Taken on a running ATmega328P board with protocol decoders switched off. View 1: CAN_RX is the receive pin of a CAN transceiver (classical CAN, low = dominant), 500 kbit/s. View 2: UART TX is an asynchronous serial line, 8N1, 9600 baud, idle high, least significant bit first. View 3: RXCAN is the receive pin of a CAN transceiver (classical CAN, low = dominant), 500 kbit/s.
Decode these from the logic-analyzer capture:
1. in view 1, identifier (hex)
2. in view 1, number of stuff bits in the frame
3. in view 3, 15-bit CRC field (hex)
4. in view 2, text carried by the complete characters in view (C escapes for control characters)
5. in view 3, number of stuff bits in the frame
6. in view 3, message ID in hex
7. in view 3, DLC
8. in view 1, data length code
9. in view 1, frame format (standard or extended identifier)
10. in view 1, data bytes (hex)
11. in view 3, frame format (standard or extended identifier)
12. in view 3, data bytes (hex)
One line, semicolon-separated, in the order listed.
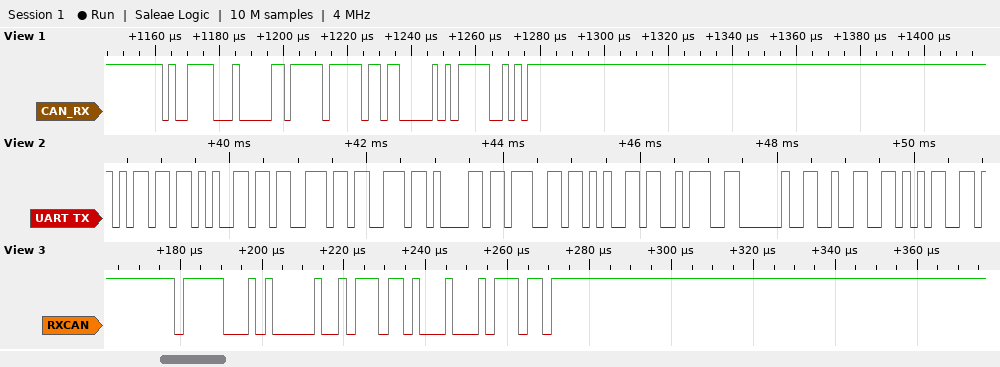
0x4F1; 5; 0x445D; "message: 25"; 2; 0x7CA; 1; 2; standard; FF F6; standard; 76
